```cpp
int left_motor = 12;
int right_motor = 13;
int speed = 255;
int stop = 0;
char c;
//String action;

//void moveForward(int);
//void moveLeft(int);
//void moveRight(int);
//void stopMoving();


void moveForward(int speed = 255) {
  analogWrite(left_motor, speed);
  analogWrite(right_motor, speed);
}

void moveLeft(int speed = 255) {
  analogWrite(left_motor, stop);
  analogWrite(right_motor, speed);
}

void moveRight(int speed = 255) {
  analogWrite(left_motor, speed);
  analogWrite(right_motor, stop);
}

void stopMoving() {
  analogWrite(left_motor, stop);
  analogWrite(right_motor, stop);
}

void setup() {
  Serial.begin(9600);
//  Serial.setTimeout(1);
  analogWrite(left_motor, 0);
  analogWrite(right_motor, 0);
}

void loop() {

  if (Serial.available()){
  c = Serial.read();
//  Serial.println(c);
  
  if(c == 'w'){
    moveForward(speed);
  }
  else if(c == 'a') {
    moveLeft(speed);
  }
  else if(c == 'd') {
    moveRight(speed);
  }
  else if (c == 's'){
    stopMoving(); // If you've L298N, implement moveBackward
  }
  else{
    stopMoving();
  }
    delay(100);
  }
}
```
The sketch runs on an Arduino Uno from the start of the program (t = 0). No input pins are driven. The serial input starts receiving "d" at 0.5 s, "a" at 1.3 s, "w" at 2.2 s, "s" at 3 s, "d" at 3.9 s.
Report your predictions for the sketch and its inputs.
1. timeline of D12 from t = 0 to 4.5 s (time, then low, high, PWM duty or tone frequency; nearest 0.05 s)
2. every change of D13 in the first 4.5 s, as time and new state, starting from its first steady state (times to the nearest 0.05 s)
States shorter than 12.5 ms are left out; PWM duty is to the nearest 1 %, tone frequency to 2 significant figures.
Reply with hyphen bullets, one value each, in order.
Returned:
- 0 s low; 0.5 s high; 1.3 s low; 2.2 s high; 3 s low; 3.9 s high
- 0 s low; 1.3 s high; 3 s low
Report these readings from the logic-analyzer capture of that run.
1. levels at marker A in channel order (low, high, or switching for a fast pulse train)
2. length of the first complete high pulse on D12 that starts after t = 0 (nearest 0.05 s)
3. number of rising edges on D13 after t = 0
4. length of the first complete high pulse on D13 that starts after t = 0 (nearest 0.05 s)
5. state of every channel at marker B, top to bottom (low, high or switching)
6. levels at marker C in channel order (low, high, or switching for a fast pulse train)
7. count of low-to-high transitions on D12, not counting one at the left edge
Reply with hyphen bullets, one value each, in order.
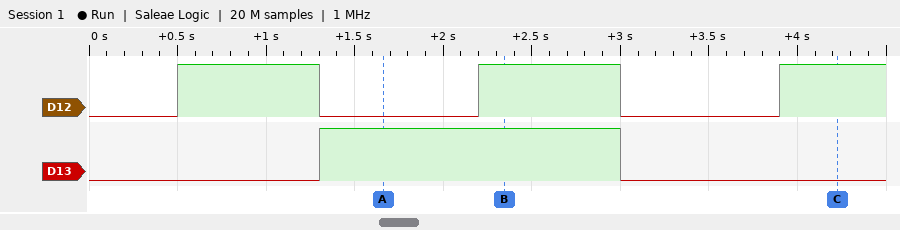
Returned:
- D12 low, D13 high
- 0.80 s
- 1
- 1.70 s
- D12 high, D13 high
- D12 high, D13 low
- 3
